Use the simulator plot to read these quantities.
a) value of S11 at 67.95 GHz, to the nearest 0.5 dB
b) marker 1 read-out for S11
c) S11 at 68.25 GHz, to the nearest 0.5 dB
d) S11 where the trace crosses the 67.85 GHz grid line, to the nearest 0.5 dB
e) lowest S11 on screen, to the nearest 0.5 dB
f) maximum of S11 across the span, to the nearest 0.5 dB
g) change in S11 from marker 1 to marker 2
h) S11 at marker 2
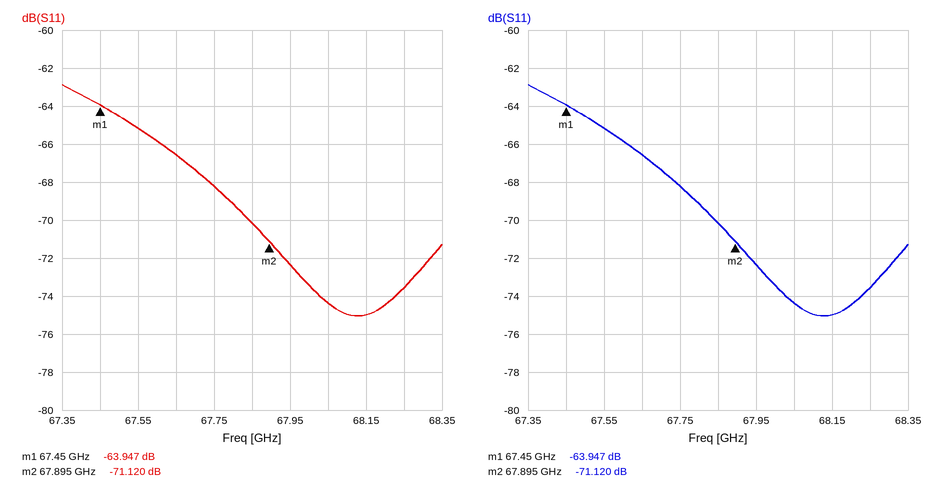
-72.5 dB
-63.947 dB
-73.5 dB
-70.0 dB
-75.0 dB
-63.0 dB
-7.173 dB
-71.120 dB
